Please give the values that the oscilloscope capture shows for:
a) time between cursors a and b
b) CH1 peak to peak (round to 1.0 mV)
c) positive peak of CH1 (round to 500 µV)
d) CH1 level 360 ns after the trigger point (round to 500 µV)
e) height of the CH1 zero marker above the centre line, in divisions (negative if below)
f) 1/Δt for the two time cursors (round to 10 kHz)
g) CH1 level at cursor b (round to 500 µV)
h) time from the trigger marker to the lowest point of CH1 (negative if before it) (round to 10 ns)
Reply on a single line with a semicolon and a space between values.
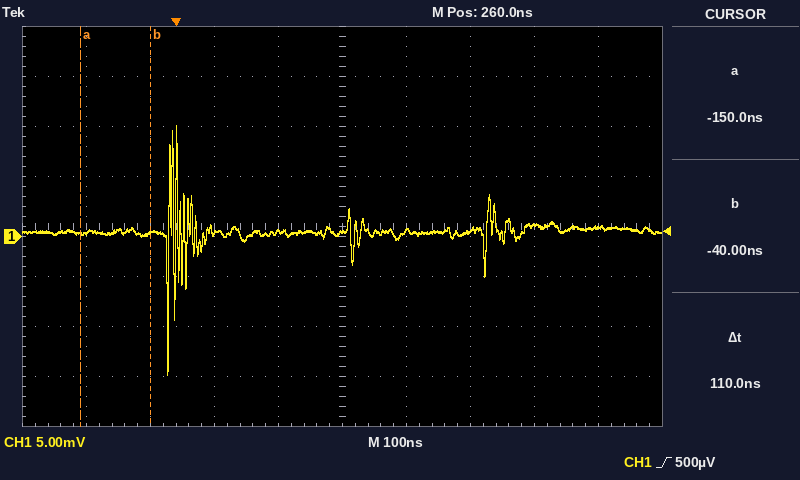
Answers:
110 ns; 25.0 mV; 11.0 mV; 500 µV; -0.2 div; 9.09 MHz; 500 µV; -10 ns
